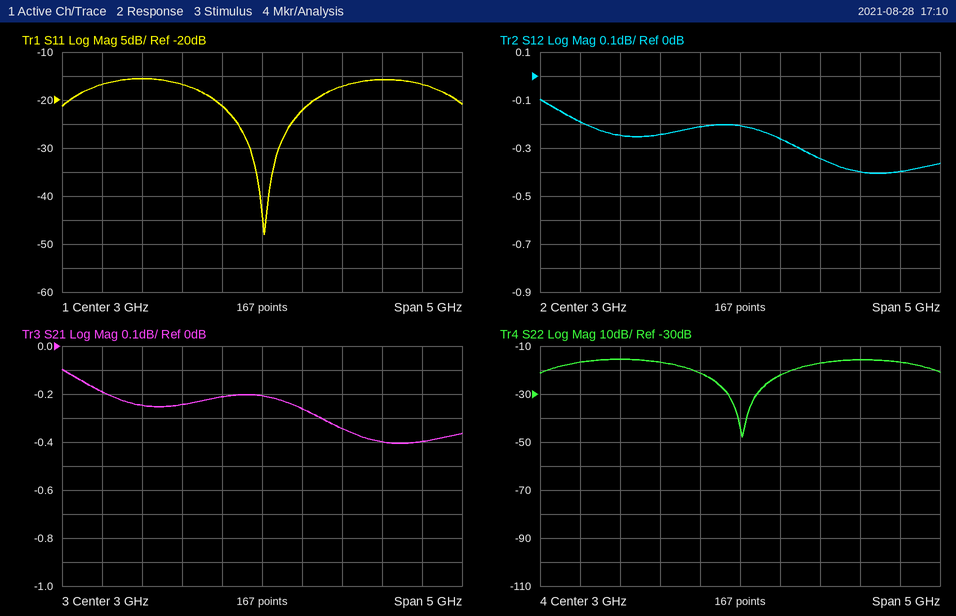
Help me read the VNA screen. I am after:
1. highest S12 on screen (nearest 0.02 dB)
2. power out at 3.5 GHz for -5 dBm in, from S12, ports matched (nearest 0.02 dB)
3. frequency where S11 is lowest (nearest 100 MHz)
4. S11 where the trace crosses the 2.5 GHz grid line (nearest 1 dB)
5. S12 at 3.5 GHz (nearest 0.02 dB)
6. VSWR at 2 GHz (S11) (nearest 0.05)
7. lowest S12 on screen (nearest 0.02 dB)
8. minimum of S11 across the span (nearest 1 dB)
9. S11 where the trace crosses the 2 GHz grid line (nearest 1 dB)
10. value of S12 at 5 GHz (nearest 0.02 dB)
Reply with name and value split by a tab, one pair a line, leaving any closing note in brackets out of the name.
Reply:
highest S12 on screen	-0.10 dB
power out at 3.5 GHz for -5 dBm in, from S12, ports matched	-5.26 dBm
frequency where S11 is lowest	3.0 GHz
S11 where the trace crosses the 2.5 GHz grid line	-21 dB
S12 at 3.5 GHz	-0.26 dB
VSWR at 2 GHz (S11)	1.35
lowest S12 on screen	-0.40 dB
minimum of S11 across the span	-48 dB
S11 where the trace crosses the 2 GHz grid line	-17 dB
value of S12 at 5 GHz	-0.40 dB
